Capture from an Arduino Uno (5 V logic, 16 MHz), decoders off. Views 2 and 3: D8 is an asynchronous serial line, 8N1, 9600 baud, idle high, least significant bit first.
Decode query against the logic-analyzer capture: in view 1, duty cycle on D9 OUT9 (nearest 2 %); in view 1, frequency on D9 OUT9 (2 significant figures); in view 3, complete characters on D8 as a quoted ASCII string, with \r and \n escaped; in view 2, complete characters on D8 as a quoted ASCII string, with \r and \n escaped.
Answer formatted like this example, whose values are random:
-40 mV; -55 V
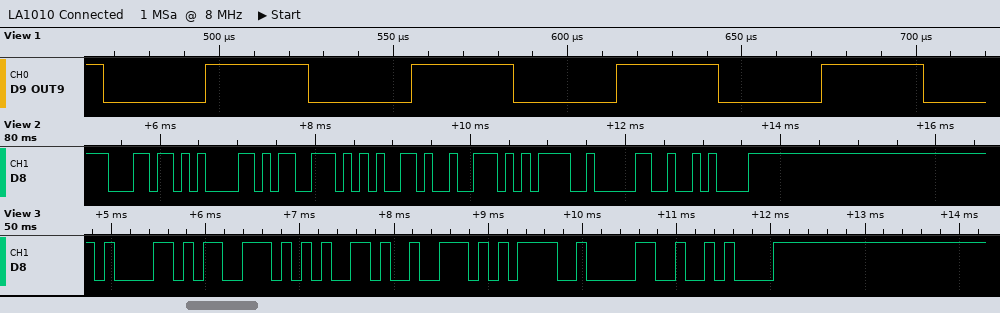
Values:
50 %; 17 kHz; "aser=0\n"; "laser=0\n"
